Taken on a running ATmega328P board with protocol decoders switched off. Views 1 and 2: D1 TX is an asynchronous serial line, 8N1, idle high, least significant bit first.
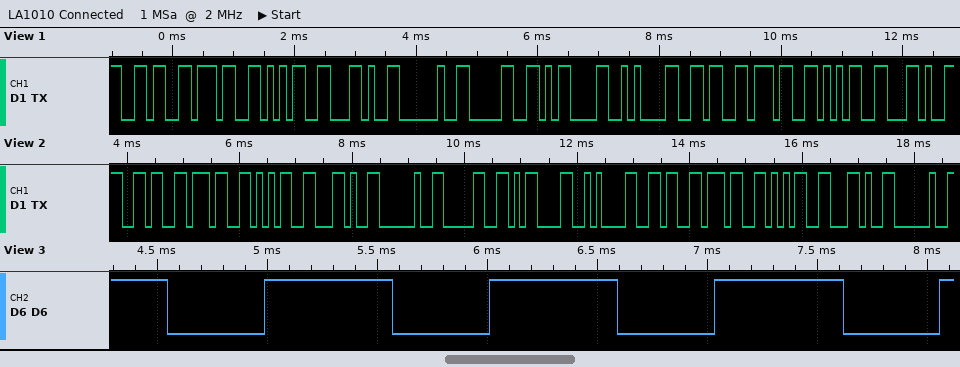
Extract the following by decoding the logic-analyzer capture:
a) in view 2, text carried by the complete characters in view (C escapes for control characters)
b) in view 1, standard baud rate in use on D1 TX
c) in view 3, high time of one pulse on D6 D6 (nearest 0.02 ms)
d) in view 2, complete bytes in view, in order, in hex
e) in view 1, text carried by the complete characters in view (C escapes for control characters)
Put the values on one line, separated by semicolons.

"675, 0\r\n675, "; 9600 baud; 0.58 ms; 36 37 35 2C 20 30 0D 0A 36 37 35 2C 20; "675, 0\r\n675,"
